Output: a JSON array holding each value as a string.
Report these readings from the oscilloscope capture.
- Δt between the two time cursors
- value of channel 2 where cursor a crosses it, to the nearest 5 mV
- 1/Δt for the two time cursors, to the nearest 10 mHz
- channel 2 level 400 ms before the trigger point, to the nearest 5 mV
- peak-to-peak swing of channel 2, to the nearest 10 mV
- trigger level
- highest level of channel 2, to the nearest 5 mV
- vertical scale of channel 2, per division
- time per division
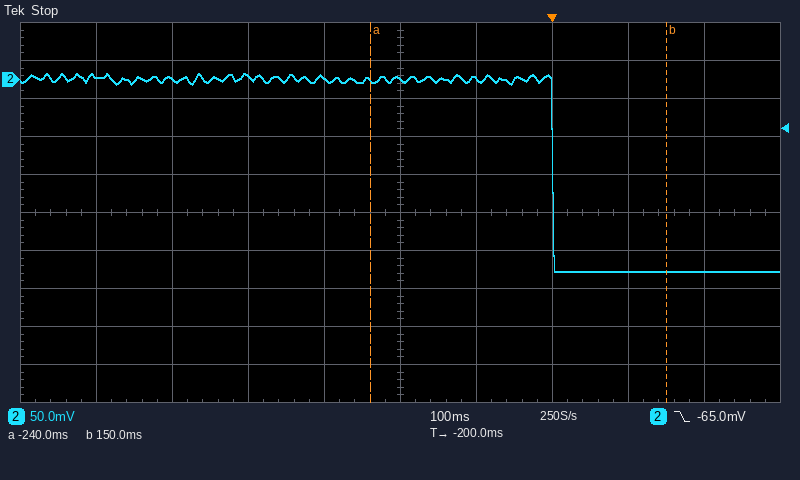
["390 ms", "0 mV", "2.56 Hz", "5 mV", "260 mV", "-65.0 mV", "10 mV", "50 mV", "100 ms"]
